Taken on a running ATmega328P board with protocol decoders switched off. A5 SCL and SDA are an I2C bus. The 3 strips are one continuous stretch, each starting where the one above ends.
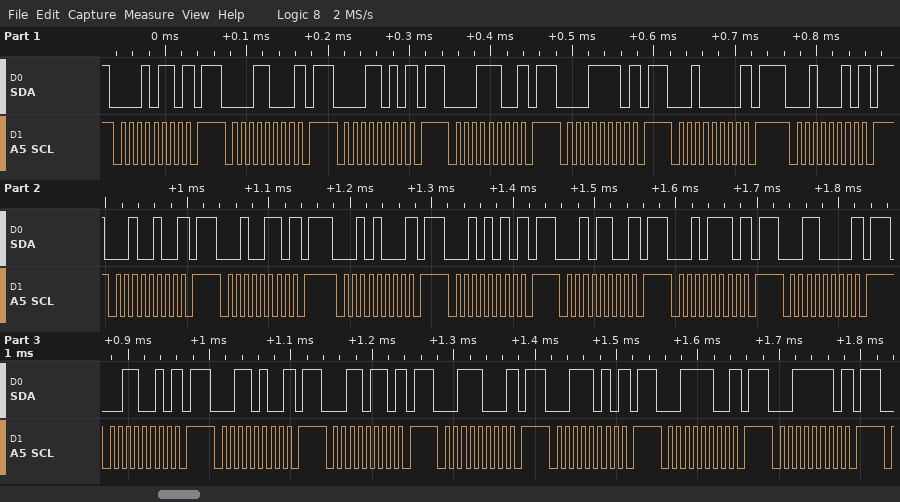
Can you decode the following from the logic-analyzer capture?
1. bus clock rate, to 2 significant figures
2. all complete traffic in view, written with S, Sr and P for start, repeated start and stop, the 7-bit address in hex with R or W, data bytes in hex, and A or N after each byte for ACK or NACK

100 kHz
S 0BW N P S 0CW N P S 0DW N P S 0EW N P S 0FW N P S 10W N P S 11W N P S 12W N P S 13W N P S 14W N P S 15W N P S 16W N P S 17W N P S 18W N P S 19W N P S 1AW N P S 1BW N P S 1CW N P S 1DW N P S 1EW N P S 1FW N P
